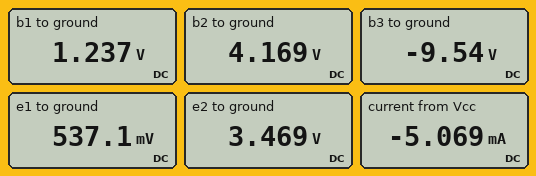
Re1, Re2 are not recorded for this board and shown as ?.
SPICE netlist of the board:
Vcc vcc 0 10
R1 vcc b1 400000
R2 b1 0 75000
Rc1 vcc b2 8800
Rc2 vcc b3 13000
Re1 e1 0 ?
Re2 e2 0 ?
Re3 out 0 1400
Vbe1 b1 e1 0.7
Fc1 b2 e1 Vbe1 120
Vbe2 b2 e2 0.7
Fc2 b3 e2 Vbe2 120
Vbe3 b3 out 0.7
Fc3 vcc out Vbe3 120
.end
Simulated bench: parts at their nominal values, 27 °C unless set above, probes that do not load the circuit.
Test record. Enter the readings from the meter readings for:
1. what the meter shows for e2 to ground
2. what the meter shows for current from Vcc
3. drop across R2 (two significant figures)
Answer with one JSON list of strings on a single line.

["3.469 V", "-5.069 mA", "1.2 V"]
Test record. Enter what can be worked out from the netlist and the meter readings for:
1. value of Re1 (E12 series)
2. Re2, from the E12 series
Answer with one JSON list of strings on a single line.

["820 Ω", "2.2 kΩ"]
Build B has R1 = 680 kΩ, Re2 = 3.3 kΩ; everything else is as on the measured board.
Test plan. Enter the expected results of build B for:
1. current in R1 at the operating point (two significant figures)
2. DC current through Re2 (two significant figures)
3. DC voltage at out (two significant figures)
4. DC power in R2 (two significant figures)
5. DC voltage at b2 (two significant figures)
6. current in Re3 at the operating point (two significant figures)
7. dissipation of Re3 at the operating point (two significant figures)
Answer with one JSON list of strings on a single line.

["13 µA", "2.2 mA", "-18 V", "10 µW", "8.0 V", "13 mA", "230 mW"]
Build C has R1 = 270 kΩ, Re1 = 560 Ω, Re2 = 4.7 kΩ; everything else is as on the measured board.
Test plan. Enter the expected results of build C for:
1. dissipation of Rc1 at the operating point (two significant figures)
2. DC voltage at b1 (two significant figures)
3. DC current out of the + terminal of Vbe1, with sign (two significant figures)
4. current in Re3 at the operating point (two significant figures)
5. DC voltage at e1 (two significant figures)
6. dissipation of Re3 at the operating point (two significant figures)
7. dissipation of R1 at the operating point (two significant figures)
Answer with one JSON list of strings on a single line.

["17 mW", "1.5 V", "-12 µA", "12 mA", "790 mV", "190 mW", "270 µW"]
